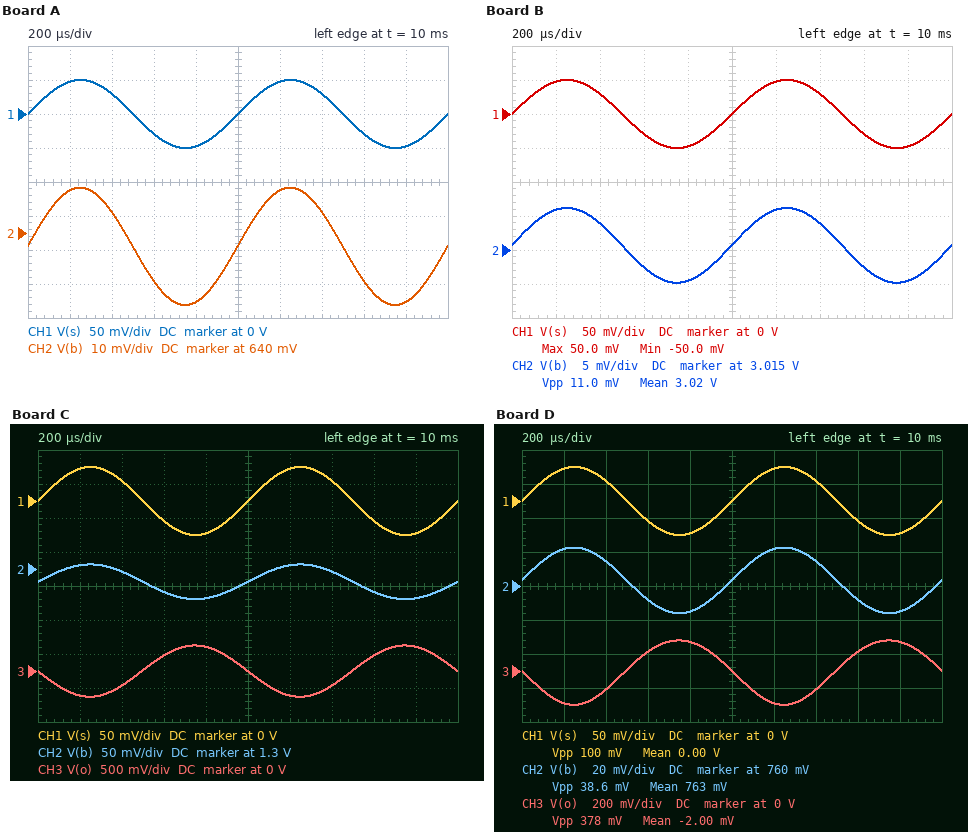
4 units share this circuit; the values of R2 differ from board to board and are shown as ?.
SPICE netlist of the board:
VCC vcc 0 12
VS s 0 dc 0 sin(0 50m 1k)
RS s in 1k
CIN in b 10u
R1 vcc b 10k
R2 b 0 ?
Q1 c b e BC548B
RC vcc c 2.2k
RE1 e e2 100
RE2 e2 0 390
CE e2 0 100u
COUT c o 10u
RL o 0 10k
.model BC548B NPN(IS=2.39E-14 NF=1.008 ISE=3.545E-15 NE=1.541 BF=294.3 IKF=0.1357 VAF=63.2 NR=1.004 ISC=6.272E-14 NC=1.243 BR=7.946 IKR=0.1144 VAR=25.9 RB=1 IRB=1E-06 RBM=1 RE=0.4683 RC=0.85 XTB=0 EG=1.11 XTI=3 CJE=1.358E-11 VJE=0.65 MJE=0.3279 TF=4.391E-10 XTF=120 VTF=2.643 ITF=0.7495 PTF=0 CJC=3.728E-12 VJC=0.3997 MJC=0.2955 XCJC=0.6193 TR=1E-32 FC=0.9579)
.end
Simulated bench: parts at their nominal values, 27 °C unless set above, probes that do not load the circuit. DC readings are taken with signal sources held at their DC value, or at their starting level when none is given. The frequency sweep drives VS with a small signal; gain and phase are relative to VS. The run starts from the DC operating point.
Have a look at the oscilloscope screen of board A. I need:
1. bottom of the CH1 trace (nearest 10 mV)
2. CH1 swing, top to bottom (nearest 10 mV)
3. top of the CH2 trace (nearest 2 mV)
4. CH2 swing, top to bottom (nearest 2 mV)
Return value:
-50 mV
100 mV
654 mV
34 mV
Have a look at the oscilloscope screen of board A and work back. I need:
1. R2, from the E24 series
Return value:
560 Ω
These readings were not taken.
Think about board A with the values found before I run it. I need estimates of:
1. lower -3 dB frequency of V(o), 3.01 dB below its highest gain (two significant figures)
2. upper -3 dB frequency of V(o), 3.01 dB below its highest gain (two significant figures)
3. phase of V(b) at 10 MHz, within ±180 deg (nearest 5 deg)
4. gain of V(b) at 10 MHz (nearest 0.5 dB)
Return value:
14 Hz
12 MHz
-30 deg
-11.5 dB
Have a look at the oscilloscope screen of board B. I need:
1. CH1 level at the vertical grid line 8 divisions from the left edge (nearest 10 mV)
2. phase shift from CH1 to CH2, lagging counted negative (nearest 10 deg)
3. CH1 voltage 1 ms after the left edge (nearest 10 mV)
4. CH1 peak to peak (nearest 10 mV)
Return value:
-30 mV
0 deg
0 V
100 mV
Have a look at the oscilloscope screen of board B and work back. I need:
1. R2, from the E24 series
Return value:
5.6 kΩ
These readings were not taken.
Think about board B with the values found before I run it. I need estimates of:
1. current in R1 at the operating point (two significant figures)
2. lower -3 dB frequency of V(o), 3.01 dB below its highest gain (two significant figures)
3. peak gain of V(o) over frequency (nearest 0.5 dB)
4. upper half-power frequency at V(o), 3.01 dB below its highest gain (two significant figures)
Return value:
900 µA
3.7 Hz
-23.0 dB
42 Hz
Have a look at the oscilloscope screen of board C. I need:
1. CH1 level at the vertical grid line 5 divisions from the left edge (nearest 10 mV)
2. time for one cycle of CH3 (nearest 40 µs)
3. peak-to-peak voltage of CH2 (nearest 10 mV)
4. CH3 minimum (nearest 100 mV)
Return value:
0 V
1.00 ms
50 mV
-400 mV
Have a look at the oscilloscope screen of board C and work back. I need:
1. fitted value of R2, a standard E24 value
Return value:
1.2 kΩ
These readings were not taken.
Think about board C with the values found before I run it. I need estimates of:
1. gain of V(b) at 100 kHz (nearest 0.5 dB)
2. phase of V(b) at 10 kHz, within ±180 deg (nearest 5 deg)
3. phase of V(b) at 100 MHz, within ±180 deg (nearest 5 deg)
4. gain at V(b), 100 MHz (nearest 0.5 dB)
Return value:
-6.0 dB
0 deg
-20 deg
-22.0 dB
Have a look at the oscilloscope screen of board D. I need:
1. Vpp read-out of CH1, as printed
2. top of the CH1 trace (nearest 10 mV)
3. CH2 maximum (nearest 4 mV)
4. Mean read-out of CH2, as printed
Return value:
100 mV
50 mV
784 mV
763 mV
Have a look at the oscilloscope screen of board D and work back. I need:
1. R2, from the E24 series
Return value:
680 Ω
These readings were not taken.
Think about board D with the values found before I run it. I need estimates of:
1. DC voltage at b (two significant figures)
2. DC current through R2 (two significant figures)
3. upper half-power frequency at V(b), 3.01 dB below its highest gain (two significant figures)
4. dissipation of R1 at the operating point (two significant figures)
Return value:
760 mV
1.1 mA
11 MHz
13 mW
